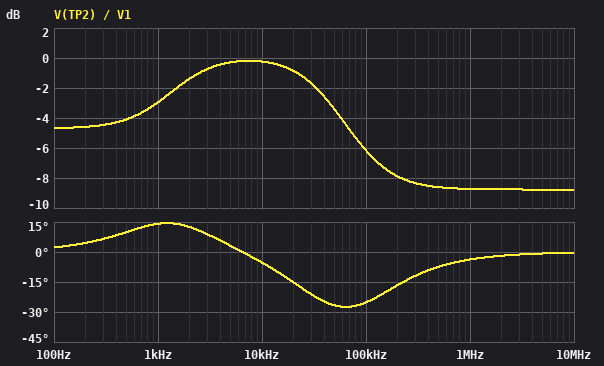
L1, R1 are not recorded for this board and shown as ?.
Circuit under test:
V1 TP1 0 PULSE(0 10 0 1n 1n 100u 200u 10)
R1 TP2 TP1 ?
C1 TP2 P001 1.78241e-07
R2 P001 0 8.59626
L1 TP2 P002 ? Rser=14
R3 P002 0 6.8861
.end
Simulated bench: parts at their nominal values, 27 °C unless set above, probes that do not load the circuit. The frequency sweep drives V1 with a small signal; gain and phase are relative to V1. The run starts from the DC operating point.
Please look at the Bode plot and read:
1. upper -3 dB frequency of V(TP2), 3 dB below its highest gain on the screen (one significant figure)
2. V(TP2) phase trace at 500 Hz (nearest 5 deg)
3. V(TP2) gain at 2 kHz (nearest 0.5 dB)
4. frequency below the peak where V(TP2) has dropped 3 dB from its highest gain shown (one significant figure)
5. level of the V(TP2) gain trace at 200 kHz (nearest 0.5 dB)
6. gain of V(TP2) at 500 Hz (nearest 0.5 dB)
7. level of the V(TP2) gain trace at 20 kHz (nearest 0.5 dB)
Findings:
50 kHz
10 deg
-1.5 dB
900 Hz
-8.0 dB
-4.0 dB
-1.0 dB
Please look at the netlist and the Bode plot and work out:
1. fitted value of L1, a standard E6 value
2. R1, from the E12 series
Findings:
3.3 mH
15 Ω
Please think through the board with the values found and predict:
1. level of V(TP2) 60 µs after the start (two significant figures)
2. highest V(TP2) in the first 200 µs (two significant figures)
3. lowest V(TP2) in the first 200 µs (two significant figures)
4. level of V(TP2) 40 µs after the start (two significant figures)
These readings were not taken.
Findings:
8.1 V
9.4 V
-2.3 V
8.7 V
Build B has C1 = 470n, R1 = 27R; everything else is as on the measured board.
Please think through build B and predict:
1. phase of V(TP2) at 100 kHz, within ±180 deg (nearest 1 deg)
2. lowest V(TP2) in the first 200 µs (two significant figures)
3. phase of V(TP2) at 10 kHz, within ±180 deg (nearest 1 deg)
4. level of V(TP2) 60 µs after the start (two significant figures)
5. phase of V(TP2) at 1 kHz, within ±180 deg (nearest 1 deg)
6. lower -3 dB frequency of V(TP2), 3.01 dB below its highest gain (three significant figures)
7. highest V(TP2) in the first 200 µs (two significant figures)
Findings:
-16 deg
-2.7 V
-27 deg
7.5 V
19 deg
1.33 kHz
8.0 V
